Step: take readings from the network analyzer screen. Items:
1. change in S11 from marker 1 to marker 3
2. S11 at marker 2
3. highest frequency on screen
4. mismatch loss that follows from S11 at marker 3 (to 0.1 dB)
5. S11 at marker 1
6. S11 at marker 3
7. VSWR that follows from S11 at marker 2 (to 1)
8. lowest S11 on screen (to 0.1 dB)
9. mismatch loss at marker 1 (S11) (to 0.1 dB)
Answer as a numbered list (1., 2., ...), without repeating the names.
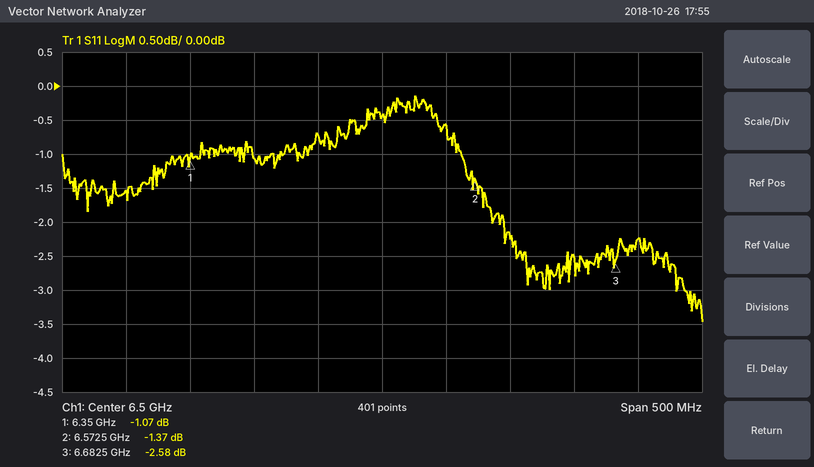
1. -1.51 dB
2. -1.37 dB
3. 6.75 GHz
4. 3.5 dB
5. -1.07 dB
6. -2.58 dB
7. 13
8. -3.5 dB
9. 6.6 dB
